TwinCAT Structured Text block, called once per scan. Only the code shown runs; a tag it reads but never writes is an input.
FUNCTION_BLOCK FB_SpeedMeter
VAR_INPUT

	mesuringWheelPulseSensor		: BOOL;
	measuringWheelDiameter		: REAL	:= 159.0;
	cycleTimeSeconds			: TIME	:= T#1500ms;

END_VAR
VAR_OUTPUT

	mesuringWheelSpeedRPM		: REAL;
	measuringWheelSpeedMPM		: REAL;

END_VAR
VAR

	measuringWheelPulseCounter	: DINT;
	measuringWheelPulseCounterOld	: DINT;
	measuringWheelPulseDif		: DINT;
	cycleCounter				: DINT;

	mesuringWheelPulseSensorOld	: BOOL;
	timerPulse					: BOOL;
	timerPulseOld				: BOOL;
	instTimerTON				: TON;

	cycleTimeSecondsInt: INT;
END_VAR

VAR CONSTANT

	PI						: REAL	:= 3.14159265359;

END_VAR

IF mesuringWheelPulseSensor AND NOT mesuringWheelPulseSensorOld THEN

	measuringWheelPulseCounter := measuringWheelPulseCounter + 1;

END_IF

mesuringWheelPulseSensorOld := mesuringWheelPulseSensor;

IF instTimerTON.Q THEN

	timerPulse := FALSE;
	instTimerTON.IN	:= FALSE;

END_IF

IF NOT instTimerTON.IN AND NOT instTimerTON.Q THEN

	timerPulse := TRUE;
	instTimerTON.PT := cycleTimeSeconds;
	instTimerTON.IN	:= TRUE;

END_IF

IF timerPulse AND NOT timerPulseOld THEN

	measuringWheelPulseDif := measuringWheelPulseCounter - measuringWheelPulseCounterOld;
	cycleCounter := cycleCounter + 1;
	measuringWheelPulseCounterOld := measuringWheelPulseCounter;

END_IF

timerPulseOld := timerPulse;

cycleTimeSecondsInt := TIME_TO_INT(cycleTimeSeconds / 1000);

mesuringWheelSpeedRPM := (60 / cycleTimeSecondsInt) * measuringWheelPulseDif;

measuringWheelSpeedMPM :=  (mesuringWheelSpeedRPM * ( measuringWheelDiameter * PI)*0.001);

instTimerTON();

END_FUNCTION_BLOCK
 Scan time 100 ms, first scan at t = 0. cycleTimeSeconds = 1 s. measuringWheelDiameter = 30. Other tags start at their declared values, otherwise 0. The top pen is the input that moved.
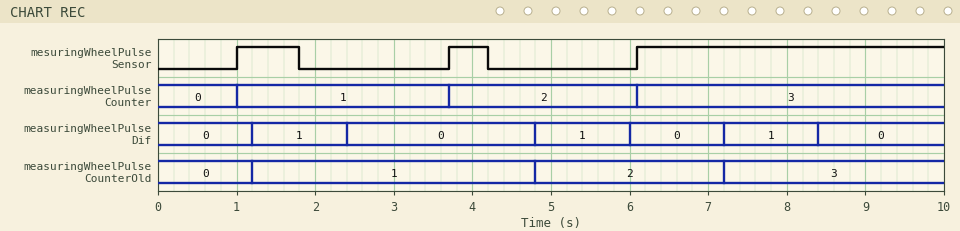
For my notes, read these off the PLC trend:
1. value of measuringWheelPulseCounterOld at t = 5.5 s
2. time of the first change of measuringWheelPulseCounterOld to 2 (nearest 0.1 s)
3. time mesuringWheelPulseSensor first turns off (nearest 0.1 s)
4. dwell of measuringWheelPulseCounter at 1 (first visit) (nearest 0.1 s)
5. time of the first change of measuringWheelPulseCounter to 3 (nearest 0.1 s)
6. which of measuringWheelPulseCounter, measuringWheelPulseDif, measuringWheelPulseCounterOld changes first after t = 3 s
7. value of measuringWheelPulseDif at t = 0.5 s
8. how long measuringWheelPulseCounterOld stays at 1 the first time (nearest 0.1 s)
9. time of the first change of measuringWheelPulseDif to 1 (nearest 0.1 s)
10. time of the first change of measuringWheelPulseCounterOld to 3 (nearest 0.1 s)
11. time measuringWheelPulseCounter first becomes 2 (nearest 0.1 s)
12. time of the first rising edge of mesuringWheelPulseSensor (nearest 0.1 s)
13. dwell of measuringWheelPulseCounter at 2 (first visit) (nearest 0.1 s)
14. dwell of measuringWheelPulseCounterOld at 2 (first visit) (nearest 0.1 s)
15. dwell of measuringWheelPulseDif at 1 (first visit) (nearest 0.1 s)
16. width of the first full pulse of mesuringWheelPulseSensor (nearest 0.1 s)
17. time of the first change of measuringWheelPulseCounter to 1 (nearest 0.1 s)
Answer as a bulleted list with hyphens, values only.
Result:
- 2
- 4.8 s
- 1.8 s
- 2.7 s
- 6.1 s
- measuringWheelPulseCounter
- 0
- 3.6 s
- 1.2 s
- 7.2 s
- 3.7 s
- 1.0 s
- 2.4 s
- 2.4 s
- 1.2 s
- 0.8 s
- 1.0 s
